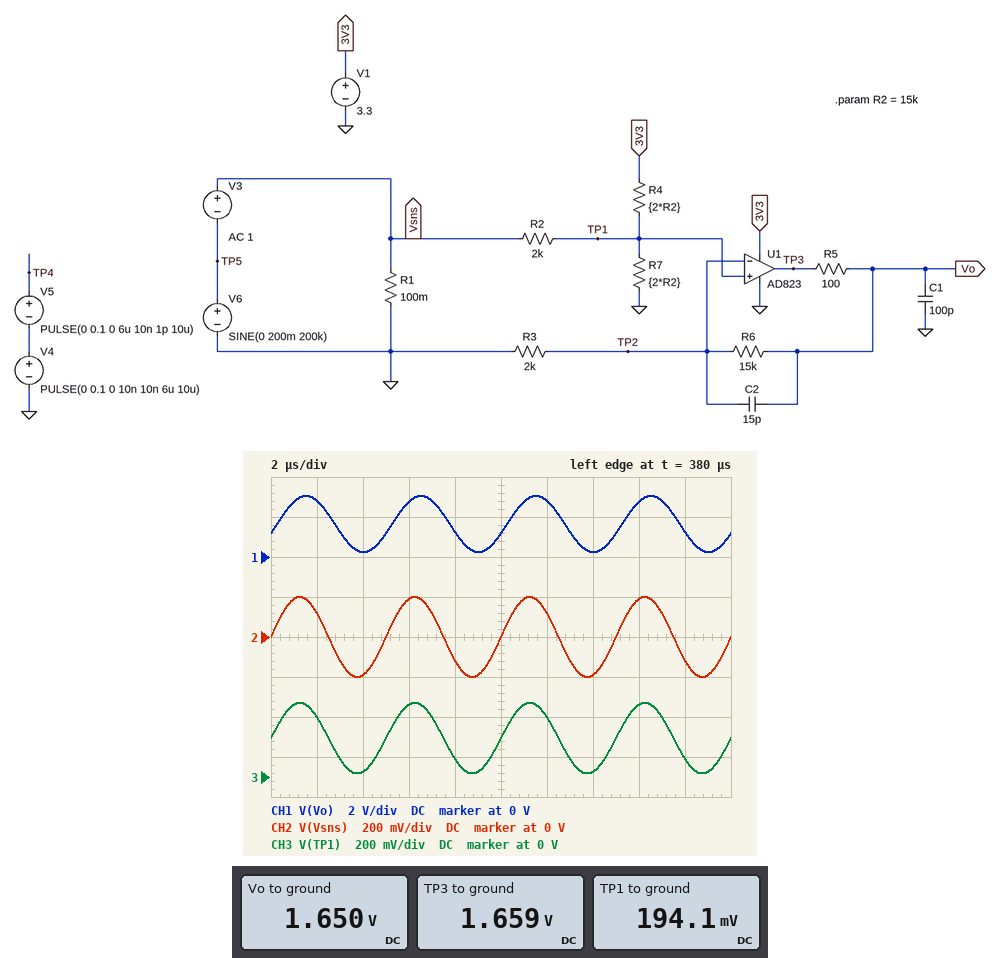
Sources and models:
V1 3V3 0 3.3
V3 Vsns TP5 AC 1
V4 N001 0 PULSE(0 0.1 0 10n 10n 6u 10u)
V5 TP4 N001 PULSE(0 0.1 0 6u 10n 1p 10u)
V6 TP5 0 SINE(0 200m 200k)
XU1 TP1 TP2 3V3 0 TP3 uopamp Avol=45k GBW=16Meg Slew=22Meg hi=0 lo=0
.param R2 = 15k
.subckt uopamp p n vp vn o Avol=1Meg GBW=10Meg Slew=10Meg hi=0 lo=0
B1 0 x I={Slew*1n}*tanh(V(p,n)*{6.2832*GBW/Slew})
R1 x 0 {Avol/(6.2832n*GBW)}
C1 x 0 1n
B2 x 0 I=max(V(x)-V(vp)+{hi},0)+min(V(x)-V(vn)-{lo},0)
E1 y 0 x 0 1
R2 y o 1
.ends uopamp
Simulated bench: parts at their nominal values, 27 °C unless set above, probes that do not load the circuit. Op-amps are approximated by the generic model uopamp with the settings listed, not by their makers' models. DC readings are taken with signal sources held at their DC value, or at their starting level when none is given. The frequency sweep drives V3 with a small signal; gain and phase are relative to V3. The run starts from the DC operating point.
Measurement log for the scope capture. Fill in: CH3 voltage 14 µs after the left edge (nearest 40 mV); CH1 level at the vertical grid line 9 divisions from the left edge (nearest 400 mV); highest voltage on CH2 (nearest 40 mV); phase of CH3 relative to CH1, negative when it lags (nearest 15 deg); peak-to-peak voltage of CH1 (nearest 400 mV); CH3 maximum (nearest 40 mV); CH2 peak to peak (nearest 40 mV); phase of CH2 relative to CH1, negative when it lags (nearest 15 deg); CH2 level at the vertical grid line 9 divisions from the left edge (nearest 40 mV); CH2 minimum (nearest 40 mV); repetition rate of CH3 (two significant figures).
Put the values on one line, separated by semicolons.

40 mV; 1.2 V; 200 mV; 15 deg; 2.8 V; 360 mV; 400 mV; 15 deg; -120 mV; -200 mV; 200 kHz
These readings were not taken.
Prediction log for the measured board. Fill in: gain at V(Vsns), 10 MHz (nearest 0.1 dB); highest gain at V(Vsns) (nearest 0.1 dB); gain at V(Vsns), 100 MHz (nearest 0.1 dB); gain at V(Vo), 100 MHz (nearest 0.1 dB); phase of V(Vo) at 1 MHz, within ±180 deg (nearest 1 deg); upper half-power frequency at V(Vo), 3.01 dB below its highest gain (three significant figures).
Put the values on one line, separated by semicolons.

0 dB; 0 dB; 0 dB; -33.0 dB; -56 deg; 536 kHz
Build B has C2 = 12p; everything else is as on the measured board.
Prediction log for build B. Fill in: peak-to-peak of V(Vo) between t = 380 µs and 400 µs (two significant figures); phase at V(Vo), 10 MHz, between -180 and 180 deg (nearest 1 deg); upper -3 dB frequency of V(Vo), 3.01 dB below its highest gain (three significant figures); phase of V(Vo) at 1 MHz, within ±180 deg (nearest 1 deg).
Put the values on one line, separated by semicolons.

2.9 V; -76 deg; 630 kHz; -54 deg
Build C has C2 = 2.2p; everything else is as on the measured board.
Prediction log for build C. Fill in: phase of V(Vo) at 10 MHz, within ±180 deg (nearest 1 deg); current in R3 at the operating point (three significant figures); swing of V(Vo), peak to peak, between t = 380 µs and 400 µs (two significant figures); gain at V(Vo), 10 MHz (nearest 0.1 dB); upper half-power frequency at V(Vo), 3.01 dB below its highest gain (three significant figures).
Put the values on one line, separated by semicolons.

-106 deg; 97.0 µA; 3.0 V; 0.2 dB; 1.48 MHz
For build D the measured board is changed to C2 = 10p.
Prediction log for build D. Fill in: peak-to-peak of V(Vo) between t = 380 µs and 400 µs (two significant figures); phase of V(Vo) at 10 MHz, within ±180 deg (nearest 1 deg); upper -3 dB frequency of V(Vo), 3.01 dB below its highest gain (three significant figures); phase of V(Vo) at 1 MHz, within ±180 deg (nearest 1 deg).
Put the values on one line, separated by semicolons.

2.9 V; -80 deg; 714 kHz; -52 deg
